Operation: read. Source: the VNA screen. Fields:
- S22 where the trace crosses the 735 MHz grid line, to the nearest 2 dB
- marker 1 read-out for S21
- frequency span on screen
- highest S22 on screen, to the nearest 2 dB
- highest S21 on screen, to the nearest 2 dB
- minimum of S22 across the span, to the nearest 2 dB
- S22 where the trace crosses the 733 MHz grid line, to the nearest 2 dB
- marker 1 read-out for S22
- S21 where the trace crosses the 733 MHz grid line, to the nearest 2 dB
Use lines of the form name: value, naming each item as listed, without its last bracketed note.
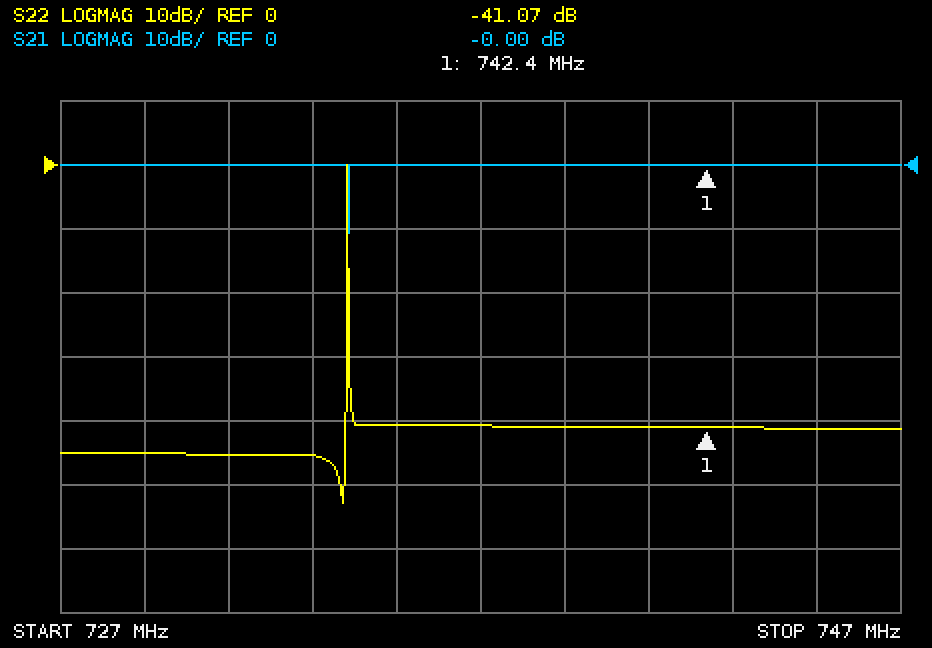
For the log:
S22 where the trace crosses the 735 MHz grid line, to the nearest 2 dB: -40 dB
marker 1 read-out for S21: -0.00 dB
frequency span on screen: 20 MHz
highest S22 on screen, to the nearest 2 dB: 0 dB
highest S21 on screen, to the nearest 2 dB: 0 dB
minimum of S22 across the span, to the nearest 2 dB: -52 dB
S22 where the trace crosses the 733 MHz grid line, to the nearest 2 dB: -46 dB
marker 1 read-out for S22: -41.07 dB
S21 where the trace crosses the 733 MHz grid line, to the nearest 2 dB: 0 dB
